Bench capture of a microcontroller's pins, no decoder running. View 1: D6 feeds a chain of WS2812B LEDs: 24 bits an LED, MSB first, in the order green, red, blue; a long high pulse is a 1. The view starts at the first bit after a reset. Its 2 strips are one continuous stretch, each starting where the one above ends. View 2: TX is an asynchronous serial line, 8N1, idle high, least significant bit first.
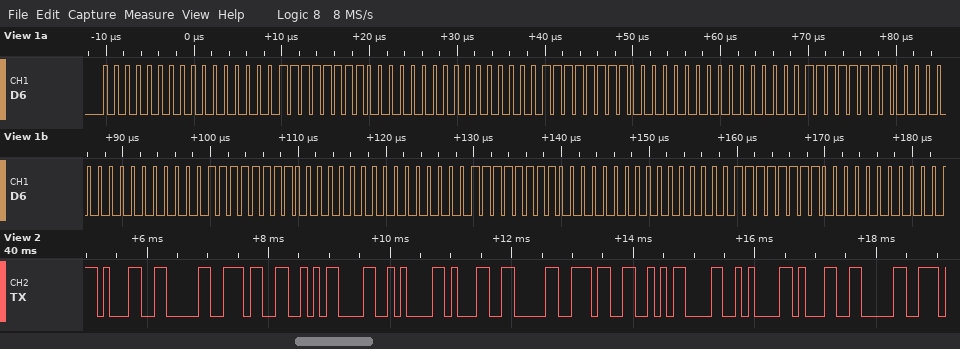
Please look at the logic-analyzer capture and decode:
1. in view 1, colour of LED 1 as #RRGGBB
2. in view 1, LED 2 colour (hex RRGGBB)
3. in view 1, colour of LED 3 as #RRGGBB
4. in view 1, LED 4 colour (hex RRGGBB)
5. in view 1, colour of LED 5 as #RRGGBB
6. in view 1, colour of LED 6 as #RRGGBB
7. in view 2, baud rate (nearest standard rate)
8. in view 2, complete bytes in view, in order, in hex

#0000FF
#0000FF
#0000FF
#0000FF
#0000FF
#0000FF
9600 baud
31 30 33 0D 0A 31 30 33 0D 0A 31 30
